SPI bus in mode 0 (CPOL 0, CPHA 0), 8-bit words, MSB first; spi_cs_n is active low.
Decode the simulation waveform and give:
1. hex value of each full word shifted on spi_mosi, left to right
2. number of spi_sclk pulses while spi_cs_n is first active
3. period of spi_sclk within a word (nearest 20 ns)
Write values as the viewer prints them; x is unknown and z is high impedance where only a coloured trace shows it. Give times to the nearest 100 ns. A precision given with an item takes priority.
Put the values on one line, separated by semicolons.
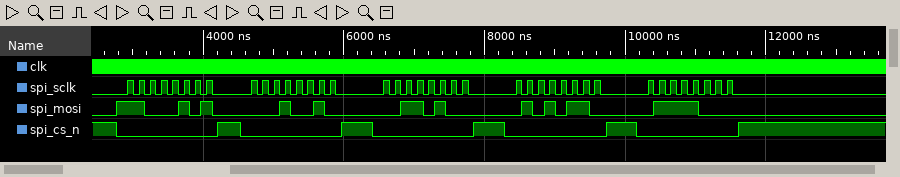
C5, 12, 34, 56, 78; 8; 160 ns
